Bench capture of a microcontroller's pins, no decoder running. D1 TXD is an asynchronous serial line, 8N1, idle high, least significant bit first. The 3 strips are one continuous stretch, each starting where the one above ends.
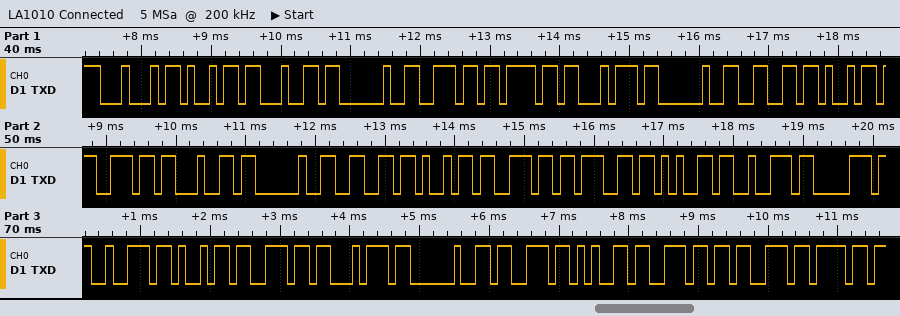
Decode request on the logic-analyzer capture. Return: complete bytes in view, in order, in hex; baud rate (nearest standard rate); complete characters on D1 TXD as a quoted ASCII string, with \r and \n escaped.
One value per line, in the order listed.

0x44 0x69 0x64 0x20 0x6E 0x6F 0x74 0x20 0x66 0x69 0x6E 0x64 0x20 0x66 0x69 0x6E 0x67 0x65 0x72 0x70 0x72 0x69 0x6E 0x74 0x20 0x73 0x65 0x6E 0x73 0x6F
9600 baud
"Did not find fingerprint senso"
